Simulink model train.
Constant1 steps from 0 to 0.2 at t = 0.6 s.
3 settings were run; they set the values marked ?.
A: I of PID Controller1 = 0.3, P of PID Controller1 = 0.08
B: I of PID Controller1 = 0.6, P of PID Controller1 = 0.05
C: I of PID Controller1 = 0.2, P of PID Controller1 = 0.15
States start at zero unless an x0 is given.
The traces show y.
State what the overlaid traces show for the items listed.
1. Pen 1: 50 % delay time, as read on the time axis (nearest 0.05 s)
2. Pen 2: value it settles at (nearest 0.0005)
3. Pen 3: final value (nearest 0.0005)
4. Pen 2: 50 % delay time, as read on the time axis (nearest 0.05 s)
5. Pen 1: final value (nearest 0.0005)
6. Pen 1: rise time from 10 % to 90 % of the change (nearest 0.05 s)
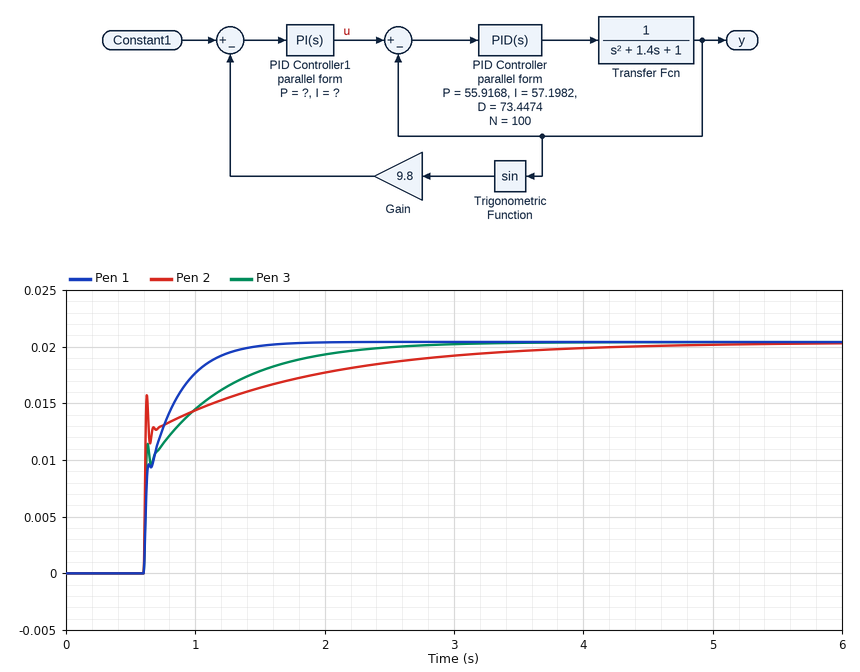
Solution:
0.70 s
0.0205
0.0205
0.60 s
0.0205
0.45 s
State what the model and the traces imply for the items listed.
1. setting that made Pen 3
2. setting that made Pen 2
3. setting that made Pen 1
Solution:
A
C
B
